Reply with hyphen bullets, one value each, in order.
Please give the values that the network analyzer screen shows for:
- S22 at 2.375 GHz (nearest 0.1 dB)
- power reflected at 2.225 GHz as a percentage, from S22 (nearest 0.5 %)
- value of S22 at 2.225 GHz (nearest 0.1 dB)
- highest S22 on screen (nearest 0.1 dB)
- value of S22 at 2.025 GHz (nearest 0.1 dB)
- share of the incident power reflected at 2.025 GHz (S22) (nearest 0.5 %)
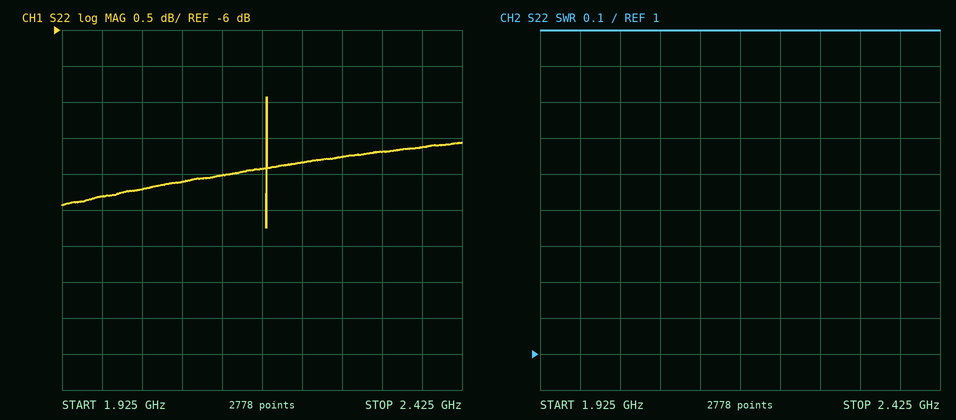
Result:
- -7.6 dB
- 16.5 %
- -7.8 dB
- -6.9 dB
- -8.2 dB
- 15.0 %
